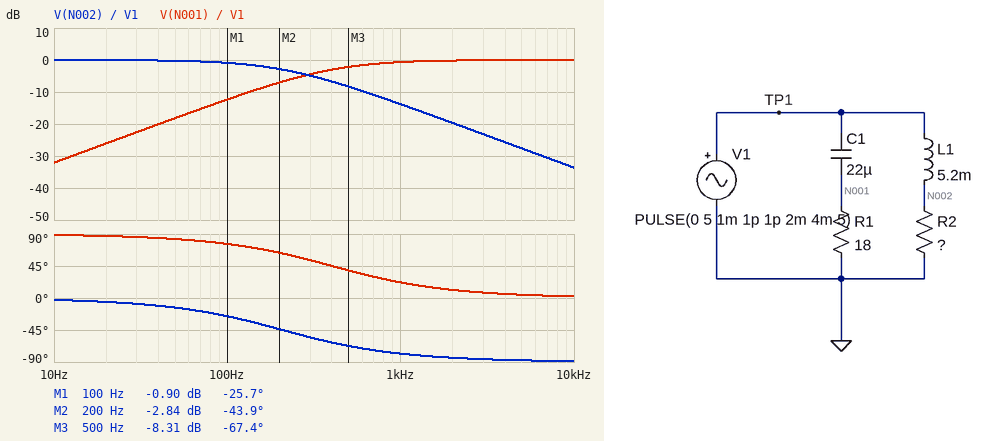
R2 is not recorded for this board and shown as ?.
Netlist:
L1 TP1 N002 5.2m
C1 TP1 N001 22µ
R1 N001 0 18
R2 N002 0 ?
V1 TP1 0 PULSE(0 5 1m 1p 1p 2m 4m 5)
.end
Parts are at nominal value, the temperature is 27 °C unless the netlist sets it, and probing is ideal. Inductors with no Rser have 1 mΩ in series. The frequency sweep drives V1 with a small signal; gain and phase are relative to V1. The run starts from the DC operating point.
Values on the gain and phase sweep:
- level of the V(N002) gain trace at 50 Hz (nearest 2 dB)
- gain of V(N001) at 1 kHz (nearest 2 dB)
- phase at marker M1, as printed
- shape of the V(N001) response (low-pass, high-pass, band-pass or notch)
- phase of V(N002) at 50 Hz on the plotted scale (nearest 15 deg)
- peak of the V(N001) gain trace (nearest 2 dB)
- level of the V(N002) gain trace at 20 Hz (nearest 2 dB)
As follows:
0 dB
0 dB
-25.7 deg
high-pass
-15 deg
0 dB
0 dB
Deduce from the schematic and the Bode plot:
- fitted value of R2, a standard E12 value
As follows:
6.8 Ω
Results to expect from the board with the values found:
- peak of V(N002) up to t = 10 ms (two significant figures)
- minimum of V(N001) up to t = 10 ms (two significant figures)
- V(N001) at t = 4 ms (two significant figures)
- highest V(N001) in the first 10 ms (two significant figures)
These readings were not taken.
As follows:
4.7 V
-5.0 V
-400 mV
5.0 V
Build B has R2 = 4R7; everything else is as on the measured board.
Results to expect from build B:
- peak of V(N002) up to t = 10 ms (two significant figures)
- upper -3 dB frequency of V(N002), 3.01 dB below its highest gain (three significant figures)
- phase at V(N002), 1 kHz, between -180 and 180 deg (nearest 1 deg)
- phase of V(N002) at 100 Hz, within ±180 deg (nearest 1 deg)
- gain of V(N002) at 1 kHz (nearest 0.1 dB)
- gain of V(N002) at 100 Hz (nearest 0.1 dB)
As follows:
4.3 V
144 Hz
-82 deg
-35 deg
-16.9 dB
-1.7 dB
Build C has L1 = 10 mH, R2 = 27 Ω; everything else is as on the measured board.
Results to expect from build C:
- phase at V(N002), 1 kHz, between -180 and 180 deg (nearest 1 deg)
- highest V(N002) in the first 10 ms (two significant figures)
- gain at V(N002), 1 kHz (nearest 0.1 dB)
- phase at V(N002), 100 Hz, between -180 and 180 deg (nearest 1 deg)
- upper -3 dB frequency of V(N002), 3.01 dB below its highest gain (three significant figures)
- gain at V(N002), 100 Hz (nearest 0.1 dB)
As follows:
-67 deg
5.0 V
-8.1 dB
-13 deg
430 Hz
-0.2 dB
